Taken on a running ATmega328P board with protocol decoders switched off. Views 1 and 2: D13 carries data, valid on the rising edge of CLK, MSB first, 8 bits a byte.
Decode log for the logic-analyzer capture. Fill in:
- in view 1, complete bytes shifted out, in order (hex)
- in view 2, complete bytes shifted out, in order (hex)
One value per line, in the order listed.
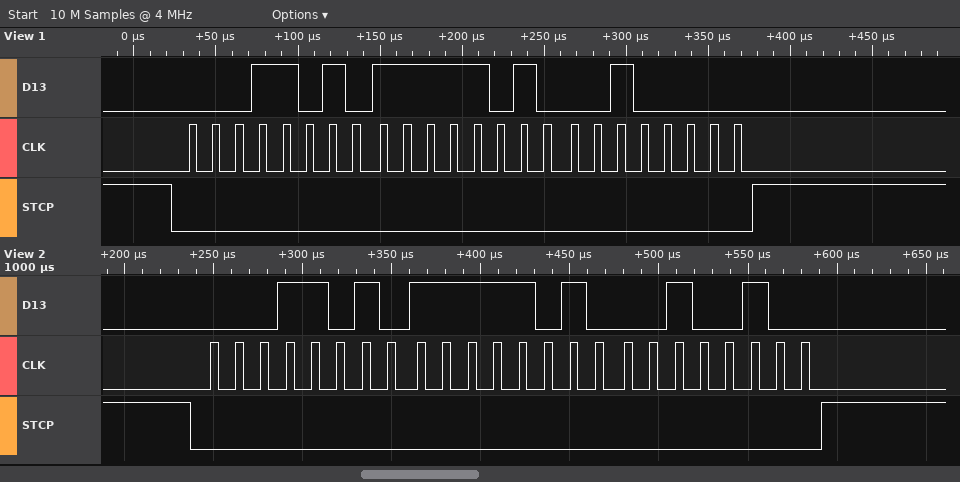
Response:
1A FA 20
1A FA 24
